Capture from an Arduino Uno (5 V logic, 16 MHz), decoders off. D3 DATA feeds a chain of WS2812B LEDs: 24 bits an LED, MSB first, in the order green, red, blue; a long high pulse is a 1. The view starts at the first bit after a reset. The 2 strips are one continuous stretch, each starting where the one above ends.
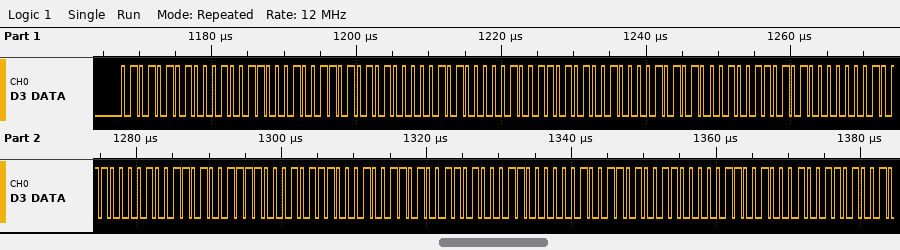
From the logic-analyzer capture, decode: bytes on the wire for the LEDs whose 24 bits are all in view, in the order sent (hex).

55 13 13 54 14 13 52 15 13 50 16 13 4F 17 13 4D 18 13 4C 19 13
